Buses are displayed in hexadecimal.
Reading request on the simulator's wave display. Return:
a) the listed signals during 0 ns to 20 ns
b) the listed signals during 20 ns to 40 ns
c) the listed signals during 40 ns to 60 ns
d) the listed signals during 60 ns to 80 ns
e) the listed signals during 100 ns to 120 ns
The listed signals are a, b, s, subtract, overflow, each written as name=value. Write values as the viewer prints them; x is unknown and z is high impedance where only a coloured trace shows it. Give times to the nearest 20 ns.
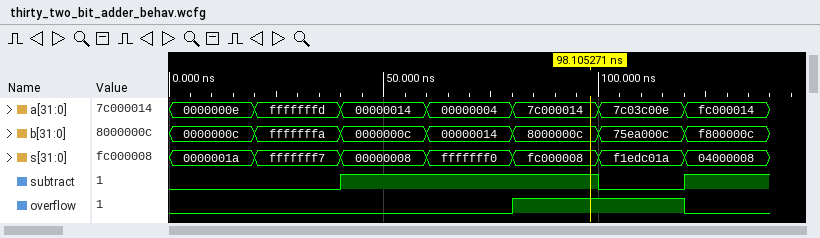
a=0000000e, b=0000000c, s=0000001a, subtract=0, overflow=0
a=fffffffd, b=fffffffa, s=fffffff7, subtract=0, overflow=0
a=00000014, b=0000000c, s=00000008, subtract=1, overflow=0
a=00000004, b=00000014, s=fffffff0, subtract=1, overflow=0
a=7c03c00e, b=75ea000c, s=f1edc01a, subtract=0, overflow=1
